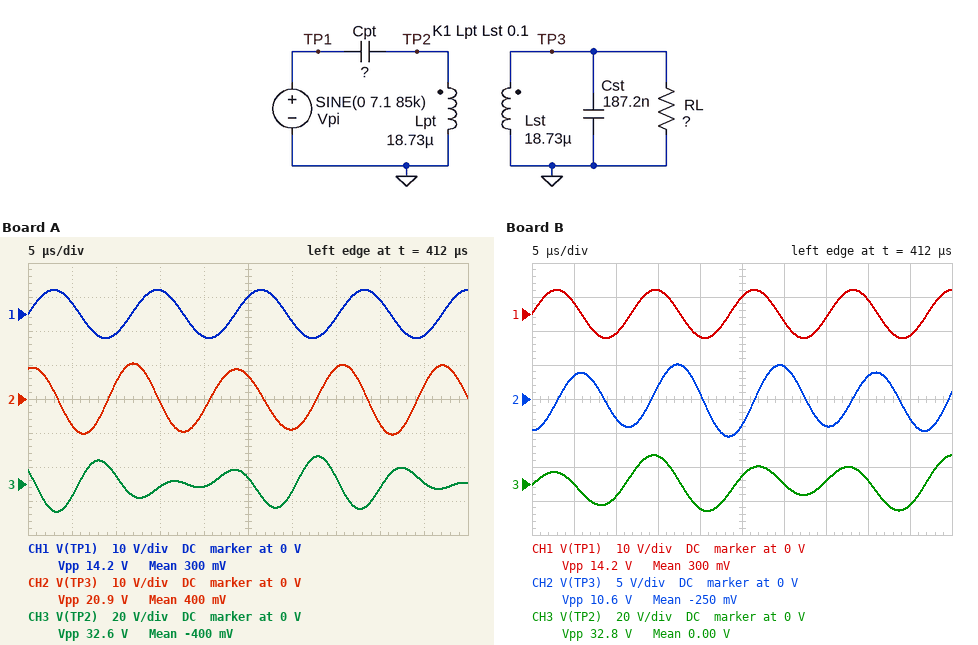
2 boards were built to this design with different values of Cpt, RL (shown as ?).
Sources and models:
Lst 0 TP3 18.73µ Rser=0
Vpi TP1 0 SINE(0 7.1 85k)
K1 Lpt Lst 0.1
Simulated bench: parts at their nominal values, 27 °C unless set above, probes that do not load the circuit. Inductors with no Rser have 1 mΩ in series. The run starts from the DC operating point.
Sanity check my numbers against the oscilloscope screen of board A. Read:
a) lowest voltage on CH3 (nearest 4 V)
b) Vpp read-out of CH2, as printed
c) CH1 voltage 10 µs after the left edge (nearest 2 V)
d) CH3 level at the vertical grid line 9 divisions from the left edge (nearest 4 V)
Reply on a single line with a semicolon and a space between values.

-16 V; 20.9 V; -6 V; 0 V
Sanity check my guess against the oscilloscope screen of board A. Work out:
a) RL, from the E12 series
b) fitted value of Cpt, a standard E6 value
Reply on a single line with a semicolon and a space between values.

120 Ω; 100 nF
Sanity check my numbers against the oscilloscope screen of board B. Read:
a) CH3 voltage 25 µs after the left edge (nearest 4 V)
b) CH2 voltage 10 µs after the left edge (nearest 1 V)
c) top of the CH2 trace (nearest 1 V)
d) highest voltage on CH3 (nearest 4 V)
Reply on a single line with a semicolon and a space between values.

4 V; -3 V; 5 V; 16 V
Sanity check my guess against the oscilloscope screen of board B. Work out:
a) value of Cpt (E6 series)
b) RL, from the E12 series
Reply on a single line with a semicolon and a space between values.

470 nF; 39 Ω
